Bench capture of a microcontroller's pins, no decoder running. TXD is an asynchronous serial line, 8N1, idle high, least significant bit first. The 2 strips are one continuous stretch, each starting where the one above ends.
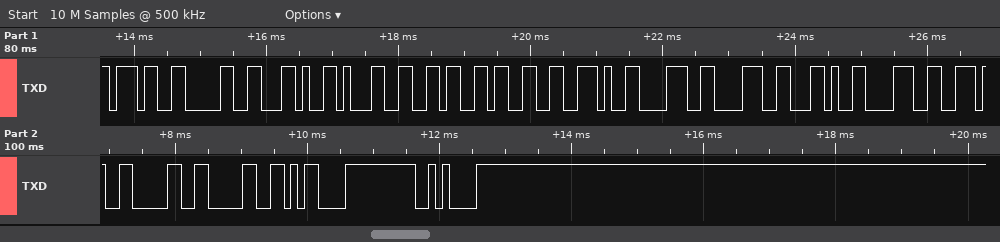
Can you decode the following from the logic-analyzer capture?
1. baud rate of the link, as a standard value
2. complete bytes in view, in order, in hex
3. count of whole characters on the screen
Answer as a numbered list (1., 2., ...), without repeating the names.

1. 9600 baud
2. 0x37 0x30 0x2C 0x31 0x36 0x33 0x2E 0x38 0x38 0x2C 0x38 0x2E 0x30 0x30 0x0D 0x0A
3. 16
